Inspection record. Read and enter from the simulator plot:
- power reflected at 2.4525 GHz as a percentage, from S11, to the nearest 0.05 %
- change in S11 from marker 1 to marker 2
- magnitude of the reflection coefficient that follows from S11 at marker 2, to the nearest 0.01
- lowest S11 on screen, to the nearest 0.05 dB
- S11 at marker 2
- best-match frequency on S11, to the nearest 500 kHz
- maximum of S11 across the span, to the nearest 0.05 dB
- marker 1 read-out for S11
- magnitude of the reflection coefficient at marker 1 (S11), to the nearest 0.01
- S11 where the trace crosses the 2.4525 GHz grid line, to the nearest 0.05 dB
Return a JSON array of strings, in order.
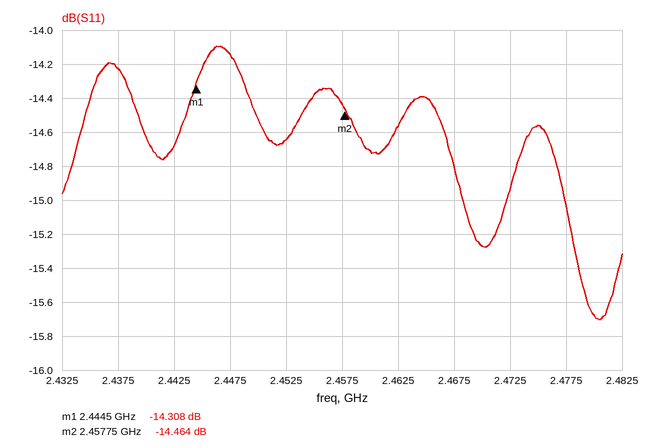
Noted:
["3.45 %", "-0.156 dB", "0.19", "-15.70 dB", "-14.464 dB", "2.4805 GHz", "-14.10 dB", "-14.308 dB", "0.19", "-14.65 dB"]
